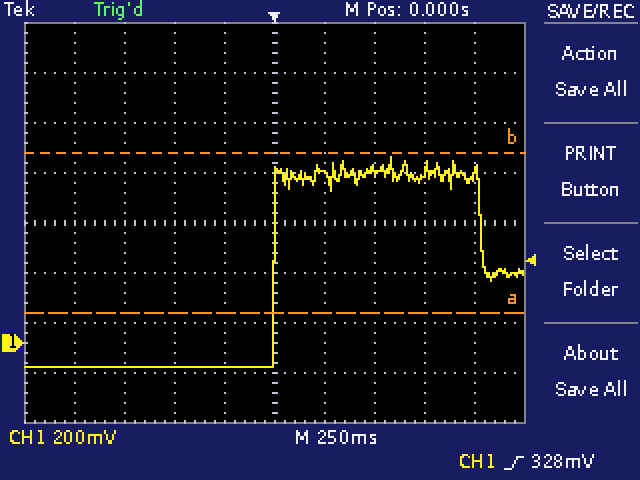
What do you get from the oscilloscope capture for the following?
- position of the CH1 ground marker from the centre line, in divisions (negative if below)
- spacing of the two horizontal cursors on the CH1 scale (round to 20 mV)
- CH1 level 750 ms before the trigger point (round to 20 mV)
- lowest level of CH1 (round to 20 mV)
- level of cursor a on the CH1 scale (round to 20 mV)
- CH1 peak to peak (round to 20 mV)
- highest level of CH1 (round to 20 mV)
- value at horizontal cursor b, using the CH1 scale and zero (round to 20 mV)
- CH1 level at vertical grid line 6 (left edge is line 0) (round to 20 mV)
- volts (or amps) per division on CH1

-2.4 div
640 mV
-100 mV
-100 mV
120 mV
840 mV
740 mV
760 mV
680 mV
200 mV
